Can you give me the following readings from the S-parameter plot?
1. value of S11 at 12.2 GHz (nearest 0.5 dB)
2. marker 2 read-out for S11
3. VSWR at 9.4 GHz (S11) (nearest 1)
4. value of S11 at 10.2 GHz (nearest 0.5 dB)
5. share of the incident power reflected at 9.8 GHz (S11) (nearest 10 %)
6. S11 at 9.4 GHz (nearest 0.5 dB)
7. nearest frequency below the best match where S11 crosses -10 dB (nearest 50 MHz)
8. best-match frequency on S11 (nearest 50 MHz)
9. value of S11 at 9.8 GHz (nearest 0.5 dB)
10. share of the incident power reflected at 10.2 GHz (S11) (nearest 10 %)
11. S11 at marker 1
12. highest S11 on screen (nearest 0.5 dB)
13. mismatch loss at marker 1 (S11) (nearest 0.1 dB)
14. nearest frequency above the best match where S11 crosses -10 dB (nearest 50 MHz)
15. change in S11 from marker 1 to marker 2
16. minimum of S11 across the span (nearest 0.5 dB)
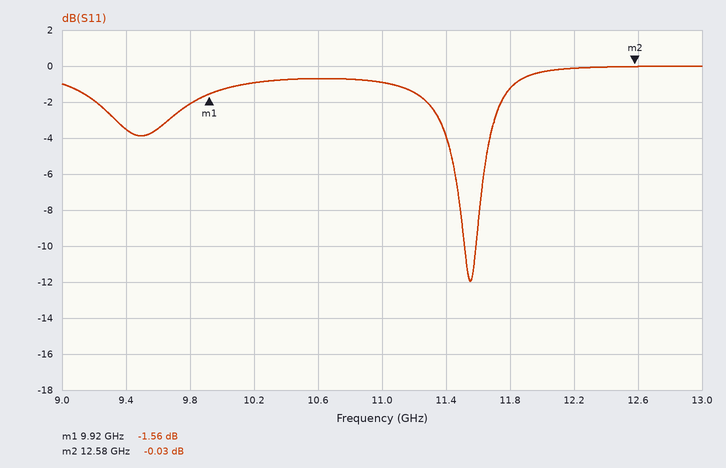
0.0 dB
-0.03 dB
5
-1.0 dB
60 %
-3.5 dB
11.50 GHz
11.55 GHz
-2.0 dB
80 %
-1.56 dB
0.0 dB
5.2 dB
11.60 GHz
1.53 dB
-12.0 dB
